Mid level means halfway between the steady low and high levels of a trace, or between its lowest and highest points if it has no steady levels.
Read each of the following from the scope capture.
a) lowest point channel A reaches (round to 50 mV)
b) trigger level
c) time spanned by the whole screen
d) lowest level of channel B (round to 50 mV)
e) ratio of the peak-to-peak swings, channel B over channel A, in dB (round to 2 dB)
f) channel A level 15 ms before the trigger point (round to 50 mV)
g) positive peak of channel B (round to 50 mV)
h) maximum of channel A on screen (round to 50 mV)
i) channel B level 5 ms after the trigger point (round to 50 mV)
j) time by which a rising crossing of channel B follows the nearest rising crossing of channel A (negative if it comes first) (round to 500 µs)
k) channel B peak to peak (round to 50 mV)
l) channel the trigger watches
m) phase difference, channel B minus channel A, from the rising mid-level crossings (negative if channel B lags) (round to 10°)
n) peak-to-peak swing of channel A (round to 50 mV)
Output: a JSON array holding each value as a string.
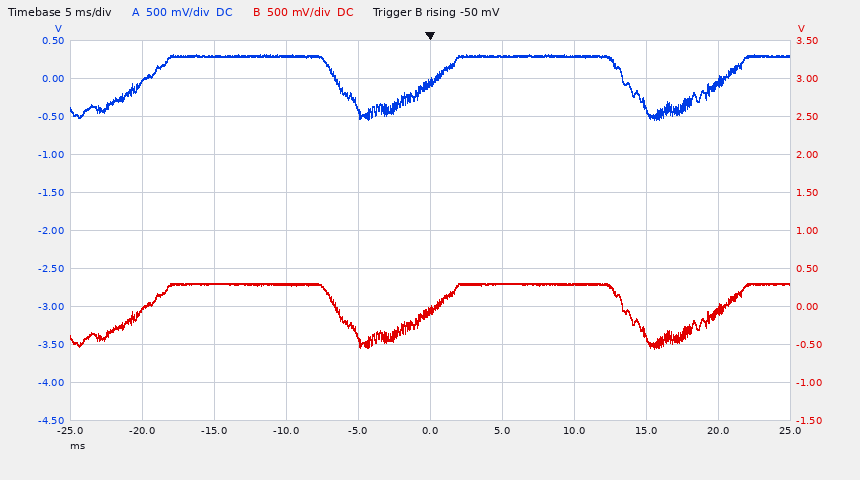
["-550 mV", "-50 mV", "50 ms", "-550 mV", "0 dB", "300 mV", "300 mV", "300 mV", "300 mV", "0.0 ms", "850 mV", "channel B", "0°", "850 mV"]
